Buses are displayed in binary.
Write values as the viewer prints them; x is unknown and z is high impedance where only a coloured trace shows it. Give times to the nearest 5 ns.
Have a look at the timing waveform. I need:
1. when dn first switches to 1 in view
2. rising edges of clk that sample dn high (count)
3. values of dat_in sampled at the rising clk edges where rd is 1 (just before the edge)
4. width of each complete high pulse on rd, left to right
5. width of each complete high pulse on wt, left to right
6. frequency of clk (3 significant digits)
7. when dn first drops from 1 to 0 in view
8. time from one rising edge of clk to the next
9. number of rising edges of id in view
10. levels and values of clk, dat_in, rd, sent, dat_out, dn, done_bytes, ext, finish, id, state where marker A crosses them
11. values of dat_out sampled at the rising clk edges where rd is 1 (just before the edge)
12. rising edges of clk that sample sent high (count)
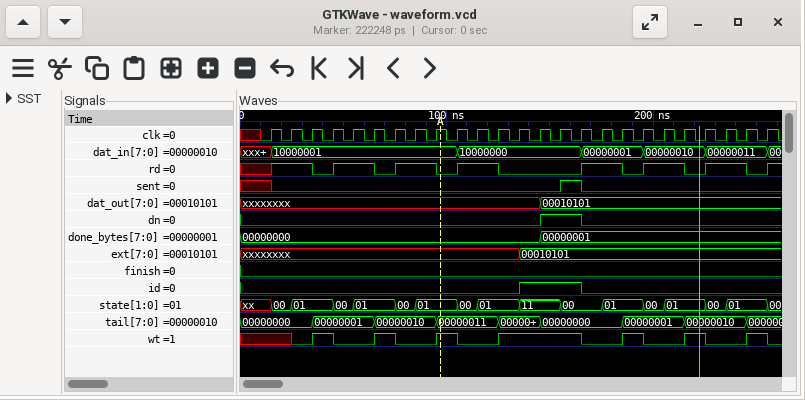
145 ns
2
10000001, 10000001, 10000001, 10000001, 10000001, 10000001, 10000000, 10000000, 00000001, 00000001, 00000010, 00000010, 00000011, 00000011
20 ns, 20 ns, 20 ns, 20 ns, 20 ns, 20 ns
10 ns, 10 ns, 10 ns, 40 ns, 10 ns, 10 ns, 10 ns
100 MHz
165 ns
10 ns
1
clk=1, dat_in=10000001, rd=0, sent=0, dat_out=xxxxxxxx, dn=0, done_bytes=00000000, ext=xxxxxxxx, finish=0, id=0, state=01
xxxxxxxx, xxxxxxxx, xxxxxxxx, xxxxxxxx, xxxxxxxx, xxxxxxxx, xxxxxxxx, xxxxxxxx, 00010101, 00010101, 00010101, 00010101, 00010101, 00010101
1
